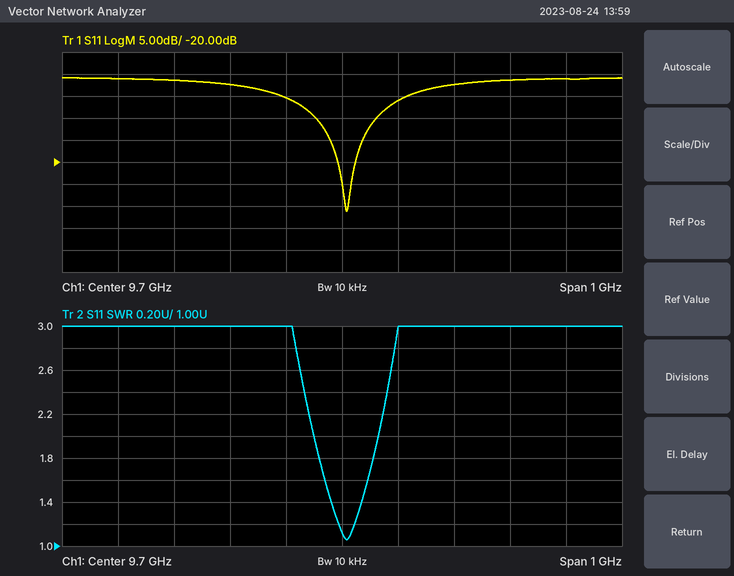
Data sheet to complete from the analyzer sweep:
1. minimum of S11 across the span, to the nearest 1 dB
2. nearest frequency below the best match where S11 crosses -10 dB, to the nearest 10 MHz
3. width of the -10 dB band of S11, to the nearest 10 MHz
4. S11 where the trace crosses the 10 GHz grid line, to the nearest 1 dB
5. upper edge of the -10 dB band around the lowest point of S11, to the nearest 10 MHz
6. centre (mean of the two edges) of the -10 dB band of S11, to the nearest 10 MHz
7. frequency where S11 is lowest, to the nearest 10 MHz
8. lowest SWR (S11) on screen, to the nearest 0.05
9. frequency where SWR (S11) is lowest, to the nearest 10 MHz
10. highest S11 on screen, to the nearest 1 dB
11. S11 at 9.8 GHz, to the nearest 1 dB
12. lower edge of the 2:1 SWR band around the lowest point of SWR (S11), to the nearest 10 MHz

-31 dB
9.65 GHz
110 MHz
-1 dB
9.76 GHz
9.71 GHz
9.71 GHz
1.05
9.71 GHz
-1 dB
-6 dB
9.65 GHz
